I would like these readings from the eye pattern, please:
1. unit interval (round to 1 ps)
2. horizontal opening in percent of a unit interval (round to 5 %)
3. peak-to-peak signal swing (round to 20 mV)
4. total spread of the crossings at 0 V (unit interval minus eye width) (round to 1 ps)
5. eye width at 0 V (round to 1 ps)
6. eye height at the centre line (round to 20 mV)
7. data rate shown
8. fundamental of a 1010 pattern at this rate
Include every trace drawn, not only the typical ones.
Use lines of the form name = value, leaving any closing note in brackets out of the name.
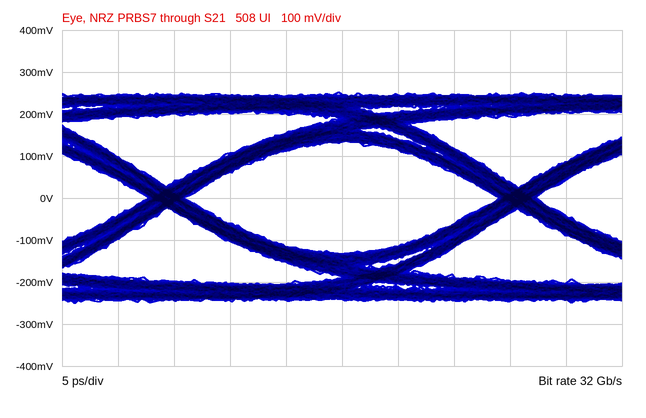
unit interval = 31 ps
horizontal opening in percent of a unit interval = 90 %
peak-to-peak signal swing = 500 mV
total spread of the crossings at 0 V (unit interval minus eye width) = 3 ps
eye width at 0 V = 28 ps
eye height at the centre line = 260 mV
data rate shown = 32 Gb/s
fundamental of a 1010 pattern at this rate = 16 GHz
